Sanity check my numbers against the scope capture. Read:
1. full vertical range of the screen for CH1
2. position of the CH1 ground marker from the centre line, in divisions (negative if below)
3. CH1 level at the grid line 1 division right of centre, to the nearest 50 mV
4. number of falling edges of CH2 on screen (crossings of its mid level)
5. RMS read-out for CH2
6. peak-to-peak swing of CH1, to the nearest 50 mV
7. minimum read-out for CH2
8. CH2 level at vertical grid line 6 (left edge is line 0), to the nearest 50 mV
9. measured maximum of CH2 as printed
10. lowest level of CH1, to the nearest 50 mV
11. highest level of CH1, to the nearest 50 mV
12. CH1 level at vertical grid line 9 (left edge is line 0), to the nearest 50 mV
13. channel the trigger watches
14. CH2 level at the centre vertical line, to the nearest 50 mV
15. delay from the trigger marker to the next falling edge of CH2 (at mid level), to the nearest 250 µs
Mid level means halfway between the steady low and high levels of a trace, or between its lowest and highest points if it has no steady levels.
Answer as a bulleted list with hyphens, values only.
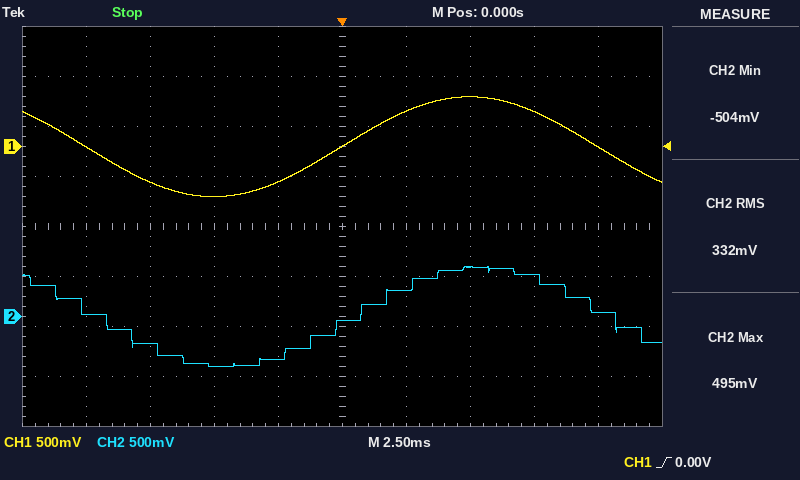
- 4 V
- +1.6 div
- 350 mV
- 2
- 332 mV
- 1.00 V
- -504 mV
- 250 mV
- 495 mV
- -500 mV
- 500 mV
- 0 mV
- CH1
- -50 mV
- 10.75 ms
